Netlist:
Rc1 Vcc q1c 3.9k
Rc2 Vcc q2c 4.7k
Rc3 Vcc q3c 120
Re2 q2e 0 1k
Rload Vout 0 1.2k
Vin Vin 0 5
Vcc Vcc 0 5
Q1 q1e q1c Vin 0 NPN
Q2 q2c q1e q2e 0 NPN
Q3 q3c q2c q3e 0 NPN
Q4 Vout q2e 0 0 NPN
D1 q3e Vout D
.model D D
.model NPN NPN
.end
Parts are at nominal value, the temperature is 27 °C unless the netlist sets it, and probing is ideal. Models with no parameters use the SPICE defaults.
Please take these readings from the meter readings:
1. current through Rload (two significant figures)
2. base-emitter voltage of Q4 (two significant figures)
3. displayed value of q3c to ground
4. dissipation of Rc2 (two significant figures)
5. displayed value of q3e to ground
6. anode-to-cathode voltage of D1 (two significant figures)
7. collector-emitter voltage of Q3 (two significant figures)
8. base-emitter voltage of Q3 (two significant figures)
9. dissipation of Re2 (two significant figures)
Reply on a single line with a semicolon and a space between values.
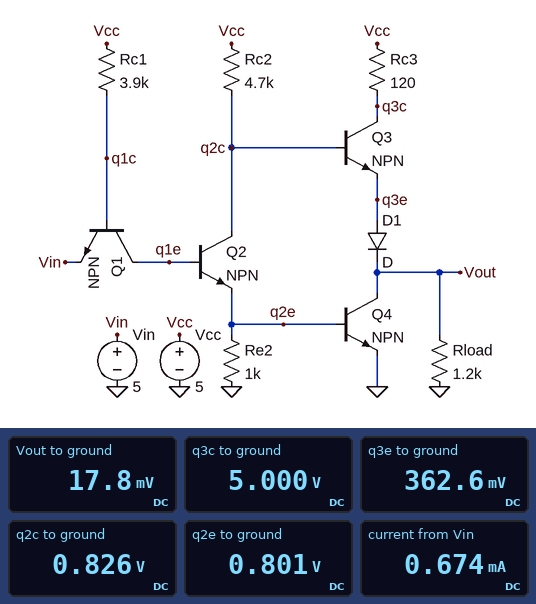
15 µA; 800 mV; 5.000 V; 3.7 mW; 362.6 mV; 340 mV; 4.6 V; 460 mV; 640 µW
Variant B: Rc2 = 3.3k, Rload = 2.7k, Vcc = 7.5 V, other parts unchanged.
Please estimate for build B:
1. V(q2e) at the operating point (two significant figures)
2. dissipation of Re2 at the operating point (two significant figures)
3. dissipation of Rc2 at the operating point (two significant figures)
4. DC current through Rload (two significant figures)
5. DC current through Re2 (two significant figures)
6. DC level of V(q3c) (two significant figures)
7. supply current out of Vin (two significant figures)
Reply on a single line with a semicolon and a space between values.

830 mV; 680 µW; 13 mW; 6.6 µA; 830 µA; 7.5 V; 1.3 mA
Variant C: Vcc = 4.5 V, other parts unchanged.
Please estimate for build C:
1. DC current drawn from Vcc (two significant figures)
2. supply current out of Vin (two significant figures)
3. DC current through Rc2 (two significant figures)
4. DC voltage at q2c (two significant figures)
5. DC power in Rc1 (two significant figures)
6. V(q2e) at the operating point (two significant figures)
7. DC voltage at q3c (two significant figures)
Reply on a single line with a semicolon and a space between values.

1.3 mA; 550 µA; 780 µA; 820 mV; 1.2 mW; 790 mV; 4.5 V
